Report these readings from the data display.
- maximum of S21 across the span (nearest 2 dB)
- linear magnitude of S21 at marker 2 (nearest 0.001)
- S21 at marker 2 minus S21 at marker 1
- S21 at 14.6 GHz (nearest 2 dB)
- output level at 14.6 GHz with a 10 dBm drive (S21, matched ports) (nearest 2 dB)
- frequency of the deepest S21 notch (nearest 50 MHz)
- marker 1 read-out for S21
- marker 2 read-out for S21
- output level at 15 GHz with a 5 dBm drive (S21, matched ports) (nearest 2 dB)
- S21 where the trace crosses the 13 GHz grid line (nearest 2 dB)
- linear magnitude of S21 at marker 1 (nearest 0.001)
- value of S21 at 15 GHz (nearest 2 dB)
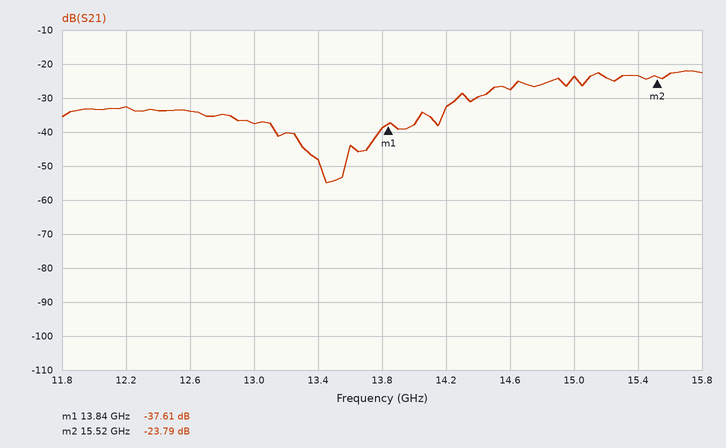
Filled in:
-22 dB
0.065
13.82 dB
-28 dB
-18 dBm
13.45 GHz
-37.61 dB
-23.79 dB
-18 dBm
-38 dB
0.013
-24 dB
